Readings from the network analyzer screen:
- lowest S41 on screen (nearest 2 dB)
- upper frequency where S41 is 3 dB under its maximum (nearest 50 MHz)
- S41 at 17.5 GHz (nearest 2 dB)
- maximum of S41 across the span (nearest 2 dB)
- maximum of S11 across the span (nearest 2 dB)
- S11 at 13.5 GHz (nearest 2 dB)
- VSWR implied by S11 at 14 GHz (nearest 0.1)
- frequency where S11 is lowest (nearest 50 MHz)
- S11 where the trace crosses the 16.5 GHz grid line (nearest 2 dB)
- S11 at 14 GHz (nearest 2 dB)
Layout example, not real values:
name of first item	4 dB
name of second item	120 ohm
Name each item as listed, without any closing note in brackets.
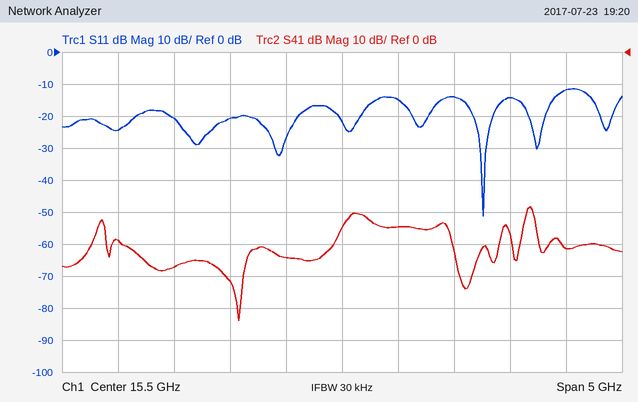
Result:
lowest S41 on screen	-84 dB
upper frequency where S41 is 3 dB under its maximum	17.20 GHz
S41 at 17.5 GHz	-62 dB
maximum of S41 across the span	-48 dB
maximum of S11 across the span	-12 dB
S11 at 13.5 GHz	-24 dB
VSWR implied by S11 at 14 GHz	1.2
frequency where S11 is lowest	16.75 GHz
S11 where the trace crosses the 16.5 GHz grid line	-14 dB
S11 at 14 GHz	-20 dB
